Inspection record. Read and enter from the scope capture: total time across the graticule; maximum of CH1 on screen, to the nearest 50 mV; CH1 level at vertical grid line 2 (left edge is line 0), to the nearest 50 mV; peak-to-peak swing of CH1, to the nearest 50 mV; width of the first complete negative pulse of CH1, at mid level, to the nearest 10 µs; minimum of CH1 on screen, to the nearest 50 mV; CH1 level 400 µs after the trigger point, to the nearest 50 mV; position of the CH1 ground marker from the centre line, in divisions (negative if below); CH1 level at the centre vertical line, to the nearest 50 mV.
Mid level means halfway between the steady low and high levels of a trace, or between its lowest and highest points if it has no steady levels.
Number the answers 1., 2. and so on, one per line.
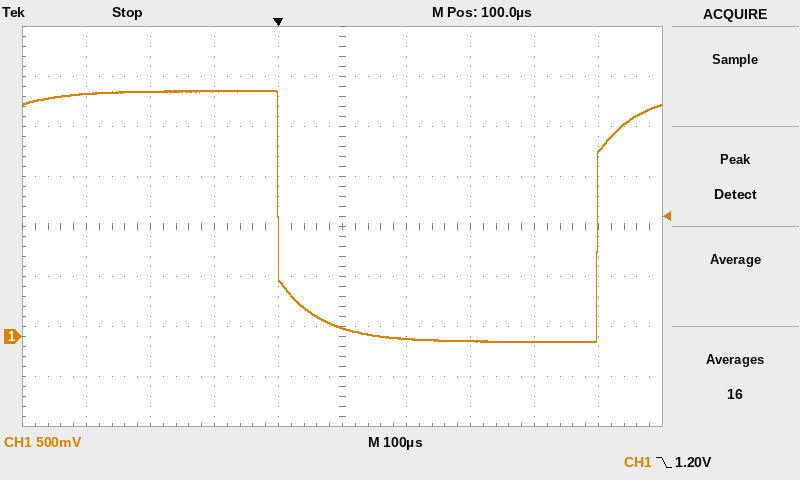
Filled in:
1. 1 ms
2. 2.45 V
3. 2.45 V
4. 2.50 V
5. 500 µs
6. -50 mV
7. -50 mV
8. -2.2 div
9. 100 mV
